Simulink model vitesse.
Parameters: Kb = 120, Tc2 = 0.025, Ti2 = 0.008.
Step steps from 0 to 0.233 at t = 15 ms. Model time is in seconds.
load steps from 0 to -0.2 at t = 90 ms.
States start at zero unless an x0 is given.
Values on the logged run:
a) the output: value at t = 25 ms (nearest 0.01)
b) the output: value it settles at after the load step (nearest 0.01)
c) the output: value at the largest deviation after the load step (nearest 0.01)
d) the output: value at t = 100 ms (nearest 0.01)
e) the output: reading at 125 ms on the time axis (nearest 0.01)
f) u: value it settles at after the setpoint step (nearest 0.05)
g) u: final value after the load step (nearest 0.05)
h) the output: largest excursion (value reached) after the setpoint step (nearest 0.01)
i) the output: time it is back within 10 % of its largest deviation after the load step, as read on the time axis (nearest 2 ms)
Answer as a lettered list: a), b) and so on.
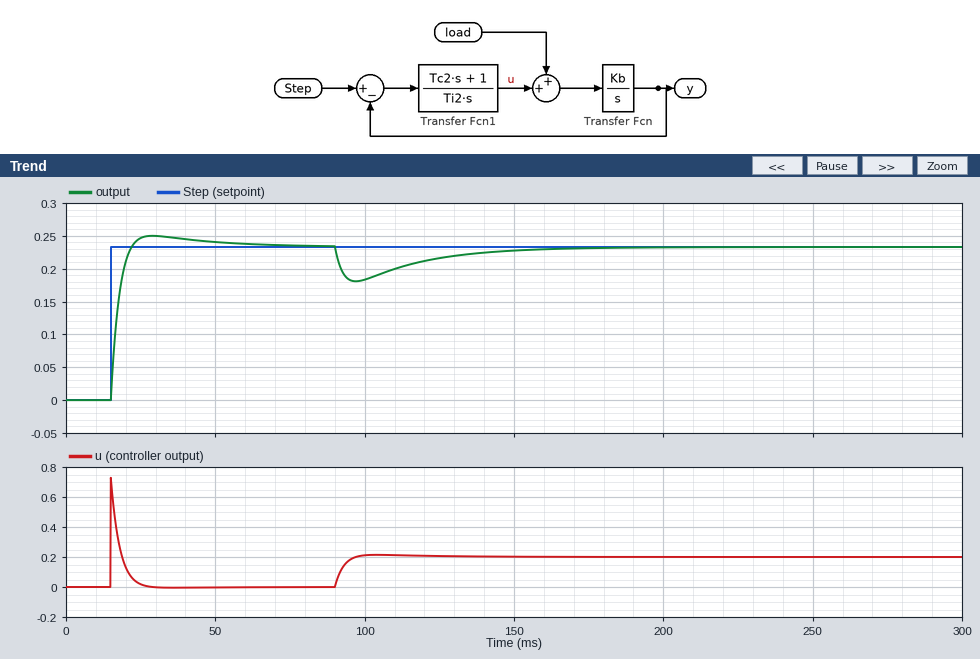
a) 0.25
b) 0.23
c) 0.18
d) 0.18
e) 0.22
f) 0.00
g) 0.20
h) 0.25
i) 150 ms
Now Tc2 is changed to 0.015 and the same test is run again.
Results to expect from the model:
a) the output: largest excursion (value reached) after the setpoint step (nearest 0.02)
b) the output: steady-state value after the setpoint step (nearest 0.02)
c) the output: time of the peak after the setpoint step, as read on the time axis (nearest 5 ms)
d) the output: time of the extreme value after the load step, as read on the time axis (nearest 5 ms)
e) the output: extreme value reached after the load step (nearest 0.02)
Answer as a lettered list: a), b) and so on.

a) 0.26
b) 0.24
c) 30 ms
d) 100 ms
e) 0.16
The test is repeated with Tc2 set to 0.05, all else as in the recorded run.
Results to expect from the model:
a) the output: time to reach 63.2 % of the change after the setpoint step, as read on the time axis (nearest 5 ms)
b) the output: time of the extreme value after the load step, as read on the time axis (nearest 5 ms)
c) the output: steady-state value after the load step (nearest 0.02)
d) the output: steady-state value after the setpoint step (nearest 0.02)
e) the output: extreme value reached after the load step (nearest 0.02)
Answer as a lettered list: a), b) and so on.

a) 15 ms
b) 95 ms
c) 0.24
d) 0.24
e) 0.20
